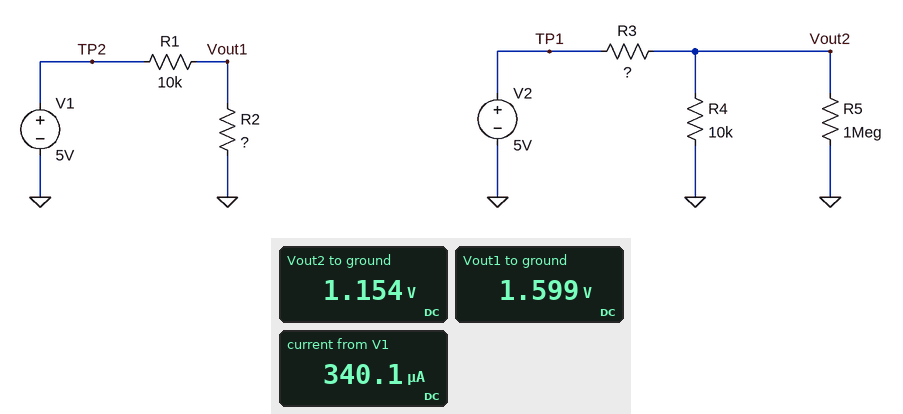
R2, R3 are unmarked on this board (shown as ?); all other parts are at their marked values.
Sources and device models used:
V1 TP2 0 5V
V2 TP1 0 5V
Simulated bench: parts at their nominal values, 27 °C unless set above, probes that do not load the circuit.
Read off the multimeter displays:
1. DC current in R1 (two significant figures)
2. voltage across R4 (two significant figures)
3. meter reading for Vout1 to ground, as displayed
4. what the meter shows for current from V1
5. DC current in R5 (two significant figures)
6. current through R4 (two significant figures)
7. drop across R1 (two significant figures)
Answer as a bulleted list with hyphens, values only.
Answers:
- 340 µA
- 1.2 V
- 1.599 V
- 340.1 µA
- 1.2 µA
- 120 µA
- 3.4 V
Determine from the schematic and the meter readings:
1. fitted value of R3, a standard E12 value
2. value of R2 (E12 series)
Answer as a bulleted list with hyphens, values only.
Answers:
- 33 kΩ
- 4.7 kΩ
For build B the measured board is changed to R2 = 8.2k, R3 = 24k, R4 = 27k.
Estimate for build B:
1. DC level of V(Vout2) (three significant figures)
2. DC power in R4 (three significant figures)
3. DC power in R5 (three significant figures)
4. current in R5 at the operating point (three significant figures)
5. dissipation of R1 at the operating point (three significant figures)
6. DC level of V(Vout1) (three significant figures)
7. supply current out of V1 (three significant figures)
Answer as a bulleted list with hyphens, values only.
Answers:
- 2.61 V
- 253 µW
- 6.83 µW
- 2.61 µA
- 755 µW
- 2.25 V
- 275 µA
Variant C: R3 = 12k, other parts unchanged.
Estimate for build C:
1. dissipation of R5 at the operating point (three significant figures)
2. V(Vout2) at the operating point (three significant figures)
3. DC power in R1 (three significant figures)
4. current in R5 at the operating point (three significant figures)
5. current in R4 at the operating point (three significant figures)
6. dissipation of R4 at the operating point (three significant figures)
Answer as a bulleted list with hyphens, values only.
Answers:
- 5.11 µW
- 2.26 V
- 1.16 mW
- 2.26 µA
- 226 µA
- 511 µW
